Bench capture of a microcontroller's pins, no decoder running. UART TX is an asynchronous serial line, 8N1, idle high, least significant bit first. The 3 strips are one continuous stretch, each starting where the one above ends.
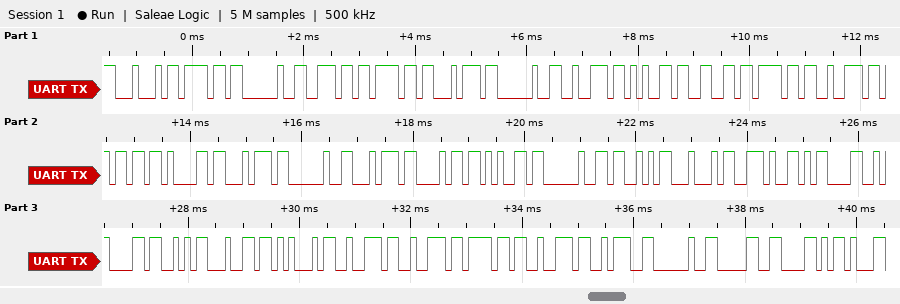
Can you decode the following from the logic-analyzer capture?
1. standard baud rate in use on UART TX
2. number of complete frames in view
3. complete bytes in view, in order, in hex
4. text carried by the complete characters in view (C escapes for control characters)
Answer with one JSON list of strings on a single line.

["9600 baud", "36", "44 6F 20 6E 6F 74 20 72 65 66 6F 72 6D 61 74 20 74 68 65 20 53 44 2E 0D 0A 53 64 45 72 72 6F 72 3A 20 30 58", "\"Do not reformat the SD.\\r\\nSdError: 0X\""]
